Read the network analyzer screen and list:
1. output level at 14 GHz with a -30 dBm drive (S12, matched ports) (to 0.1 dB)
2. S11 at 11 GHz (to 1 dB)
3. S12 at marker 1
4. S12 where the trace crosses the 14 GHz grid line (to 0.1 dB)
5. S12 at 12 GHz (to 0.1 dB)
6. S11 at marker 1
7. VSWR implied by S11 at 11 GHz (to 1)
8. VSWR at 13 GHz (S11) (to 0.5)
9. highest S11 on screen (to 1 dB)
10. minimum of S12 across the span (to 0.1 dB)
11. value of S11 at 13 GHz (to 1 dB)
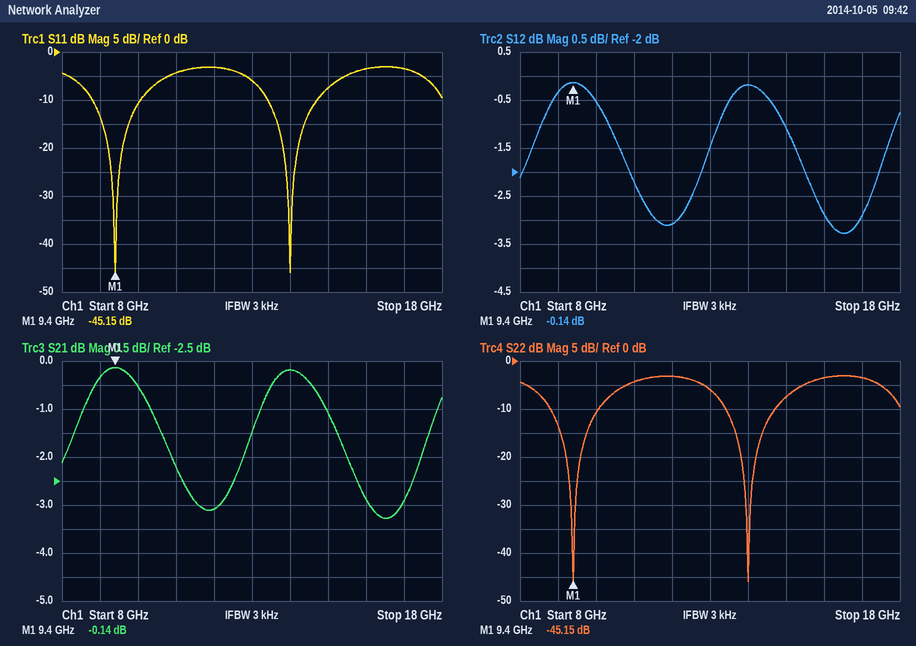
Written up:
-30.2 dBm
-4 dB
-0.14 dB
-0.2 dB
-3.1 dB
-45.15 dB
4
3.0
-3 dB
-3.3 dB
-6 dB
